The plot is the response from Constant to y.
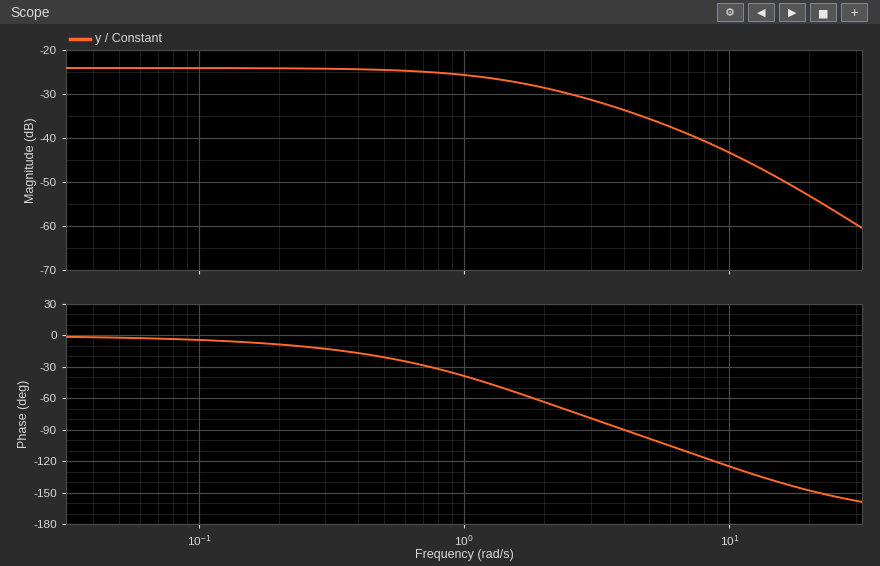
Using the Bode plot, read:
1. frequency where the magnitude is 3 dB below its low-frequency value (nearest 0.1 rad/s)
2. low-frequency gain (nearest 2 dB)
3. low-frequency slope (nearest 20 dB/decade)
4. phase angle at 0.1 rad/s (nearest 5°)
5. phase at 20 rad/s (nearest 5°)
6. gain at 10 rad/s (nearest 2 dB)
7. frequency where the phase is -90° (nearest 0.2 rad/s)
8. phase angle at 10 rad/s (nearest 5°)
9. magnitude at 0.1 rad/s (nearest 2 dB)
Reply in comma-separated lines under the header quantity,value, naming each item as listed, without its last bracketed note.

quantity,value
frequency where the magnitude is 3 dB below its low-frequency value,1.5 rad/s
low-frequency gain,-24 dB
low-frequency slope,0 dB/decade
phase angle at 0.1 rad/s,-5°
phase at 20 rad/s,-150°
gain at 10 rad/s,-44 dB
frequency where the phase is -90°,4.0 rad/s
phase angle at 10 rad/s,-125°
magnitude at 0.1 rad/s,-24 dB
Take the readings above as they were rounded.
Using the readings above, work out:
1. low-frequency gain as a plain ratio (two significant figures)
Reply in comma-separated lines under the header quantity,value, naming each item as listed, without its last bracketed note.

quantity,value
low-frequency gain as a plain ratio,0.063
